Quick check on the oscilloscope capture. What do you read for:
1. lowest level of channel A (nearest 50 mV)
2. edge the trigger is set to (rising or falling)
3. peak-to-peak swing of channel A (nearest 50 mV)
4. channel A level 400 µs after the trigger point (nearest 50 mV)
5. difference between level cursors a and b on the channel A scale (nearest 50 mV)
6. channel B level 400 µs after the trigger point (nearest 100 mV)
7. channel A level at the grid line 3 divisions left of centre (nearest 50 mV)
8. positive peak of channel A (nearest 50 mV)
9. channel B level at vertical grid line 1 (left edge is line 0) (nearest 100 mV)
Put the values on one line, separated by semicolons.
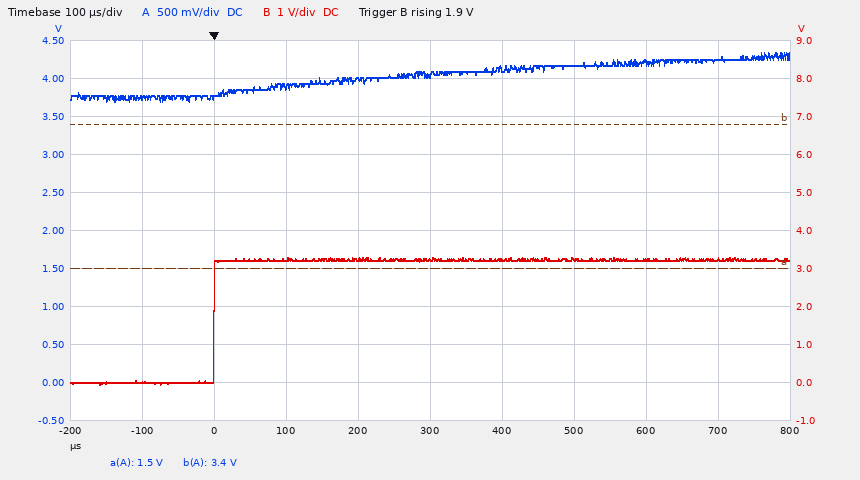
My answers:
3.70 V; rising; 650 mV; 4.15 V; 1.90 V; 3.2 V; 3.75 V; 4.35 V; 0.0 V
